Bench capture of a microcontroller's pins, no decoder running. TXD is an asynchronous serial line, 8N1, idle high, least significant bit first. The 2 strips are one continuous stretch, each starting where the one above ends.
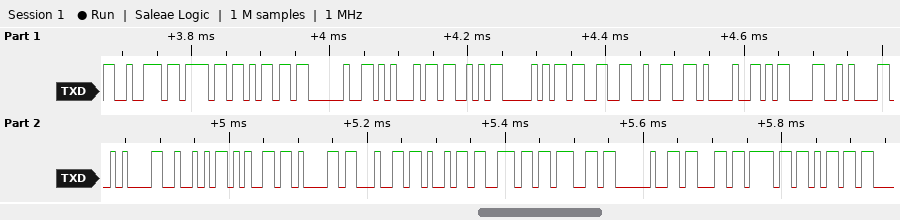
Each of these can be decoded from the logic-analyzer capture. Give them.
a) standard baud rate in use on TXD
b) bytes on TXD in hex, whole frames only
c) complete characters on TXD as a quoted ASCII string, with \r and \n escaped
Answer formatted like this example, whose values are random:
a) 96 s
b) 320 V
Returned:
a) 115200 baud
b) 0x72 0x6F 0x6D 0x20 0x45 0x53 0x50 0x33 0x32 0x21 0x0D 0x0A 0x0A 0x52 0x65 0x61 0x64 0x69 0x6E 0x67 0x20 0x63 0x6F 0x6D
c) "rom ESP32!\r\n\nReading com"
